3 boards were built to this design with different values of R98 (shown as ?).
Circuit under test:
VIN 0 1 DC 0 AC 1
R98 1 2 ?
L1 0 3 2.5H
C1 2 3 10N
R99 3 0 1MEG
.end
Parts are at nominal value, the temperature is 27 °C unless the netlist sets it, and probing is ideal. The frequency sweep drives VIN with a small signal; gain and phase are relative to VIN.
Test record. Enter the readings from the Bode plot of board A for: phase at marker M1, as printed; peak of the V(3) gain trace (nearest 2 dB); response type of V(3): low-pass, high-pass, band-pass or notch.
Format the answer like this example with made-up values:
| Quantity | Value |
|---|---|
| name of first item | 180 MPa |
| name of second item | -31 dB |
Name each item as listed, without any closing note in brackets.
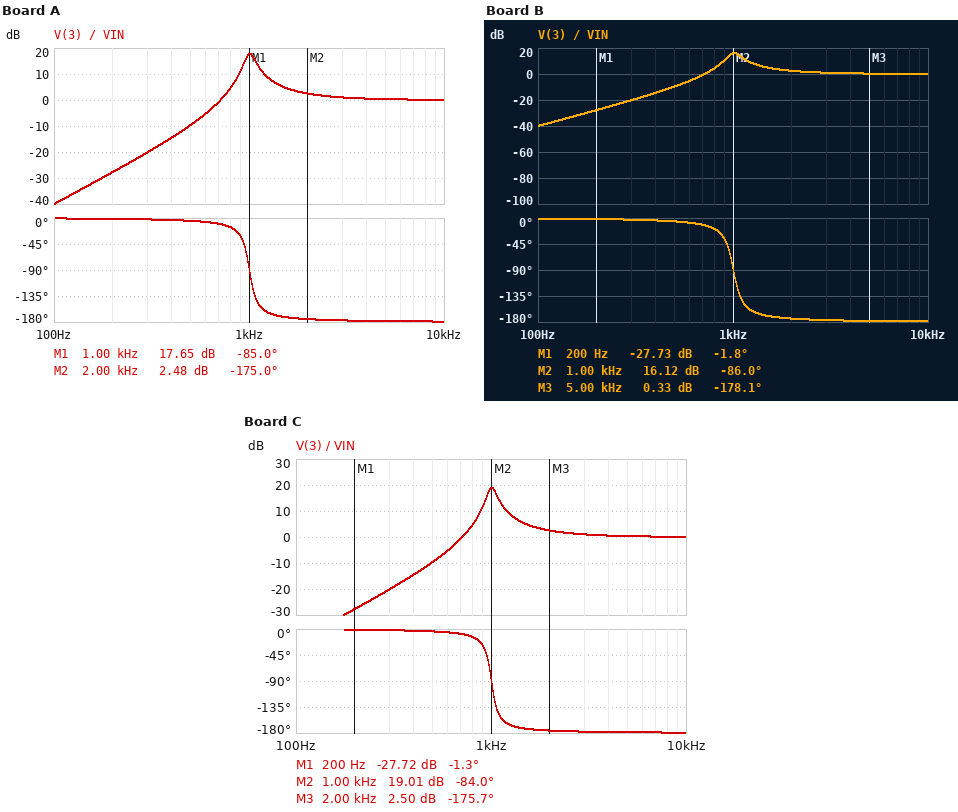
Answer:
| Quantity | Value |
|---|---|
| phase at marker M1, as printed | -85.0 deg |
| peak of the V(3) gain trace | 18 dB |
| response type of V(3): low-pass, high-pass, band-pass or notch | high-pass |
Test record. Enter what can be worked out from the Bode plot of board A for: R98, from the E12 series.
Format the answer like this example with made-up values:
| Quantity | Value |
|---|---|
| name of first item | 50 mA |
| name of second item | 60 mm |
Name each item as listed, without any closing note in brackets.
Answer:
| Quantity | Value |
|---|---|
| R98, from the E12 series | 1.8 kΩ |
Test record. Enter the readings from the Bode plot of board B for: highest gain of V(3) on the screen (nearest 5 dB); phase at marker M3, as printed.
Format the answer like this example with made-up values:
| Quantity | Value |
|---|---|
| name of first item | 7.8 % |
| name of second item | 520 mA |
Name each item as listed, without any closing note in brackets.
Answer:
| Quantity | Value |
|---|---|
| highest gain of V(3) on the screen | 15 dB |
| phase at marker M3, as printed | -178.1 deg |
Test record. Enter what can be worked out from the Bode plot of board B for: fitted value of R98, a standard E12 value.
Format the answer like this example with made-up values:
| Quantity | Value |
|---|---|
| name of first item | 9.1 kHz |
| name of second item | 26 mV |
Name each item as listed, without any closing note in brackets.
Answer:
| Quantity | Value |
|---|---|
| fitted value of R98, a standard E12 value | 2.2 kΩ |
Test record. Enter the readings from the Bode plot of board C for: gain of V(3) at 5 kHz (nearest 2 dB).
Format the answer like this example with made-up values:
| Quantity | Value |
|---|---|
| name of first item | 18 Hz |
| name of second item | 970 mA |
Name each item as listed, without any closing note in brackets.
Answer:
| Quantity | Value |
|---|---|
| gain of V(3) at 5 kHz | 0 dB |
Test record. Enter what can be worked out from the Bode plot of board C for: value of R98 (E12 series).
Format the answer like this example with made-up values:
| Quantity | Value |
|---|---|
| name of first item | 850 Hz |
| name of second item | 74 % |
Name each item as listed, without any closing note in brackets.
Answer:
| Quantity | Value |
|---|---|
| value of R98 | 1.5 kΩ |
